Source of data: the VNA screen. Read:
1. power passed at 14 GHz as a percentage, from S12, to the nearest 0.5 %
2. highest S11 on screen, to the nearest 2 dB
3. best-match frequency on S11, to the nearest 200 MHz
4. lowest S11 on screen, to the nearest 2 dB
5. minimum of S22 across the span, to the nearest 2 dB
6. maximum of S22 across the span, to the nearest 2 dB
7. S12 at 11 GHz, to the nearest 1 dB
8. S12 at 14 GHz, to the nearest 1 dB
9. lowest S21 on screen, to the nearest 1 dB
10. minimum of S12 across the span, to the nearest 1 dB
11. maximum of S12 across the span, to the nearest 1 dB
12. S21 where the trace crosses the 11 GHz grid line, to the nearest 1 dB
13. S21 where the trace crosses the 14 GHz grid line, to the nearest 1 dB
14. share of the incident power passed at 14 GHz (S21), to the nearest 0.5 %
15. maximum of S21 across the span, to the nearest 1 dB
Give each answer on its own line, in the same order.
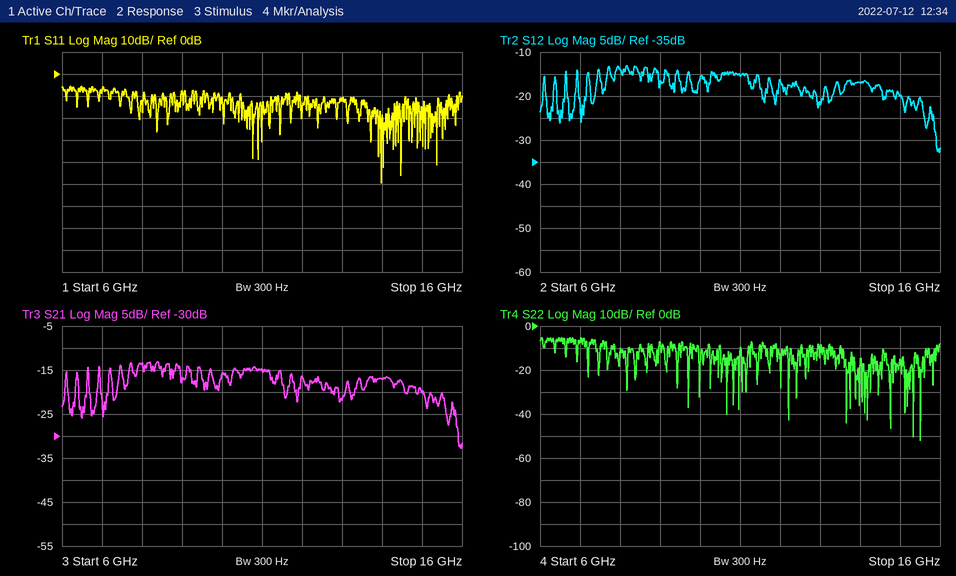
2.0 %
-6 dB
14.0 GHz
-50 dB
-52 dB
-6 dB
-15 dB
-17 dB
-33 dB
-33 dB
-13 dB
-15 dB
-17 dB
2.0 %
-13 dB
